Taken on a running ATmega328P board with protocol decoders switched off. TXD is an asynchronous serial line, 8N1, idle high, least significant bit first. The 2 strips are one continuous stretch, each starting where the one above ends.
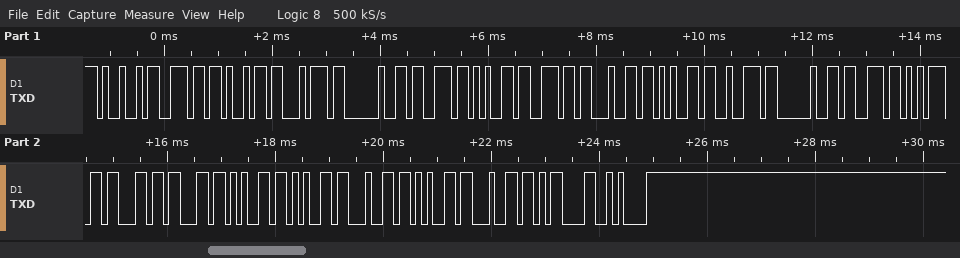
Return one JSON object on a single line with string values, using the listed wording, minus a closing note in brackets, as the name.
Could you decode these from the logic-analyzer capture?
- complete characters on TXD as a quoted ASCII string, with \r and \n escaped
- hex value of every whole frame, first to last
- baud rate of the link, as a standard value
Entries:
{"complete characters on TXD as a quoted ASCII string, with \\r and \\n escaped": "\"Init sender succeeded\\r\\n\"", "hex value of every whole frame, first to last": "0x49 0x6E 0x69 0x74 0x20 0x73 0x65 0x6E 0x64 0x65 0x72 0x20 0x73 0x75 0x63 0x63 0x65 0x65 0x64 0x65 0x64 0x0D 0x0A", "baud rate of the link, as a standard value": "9600 baud"}
